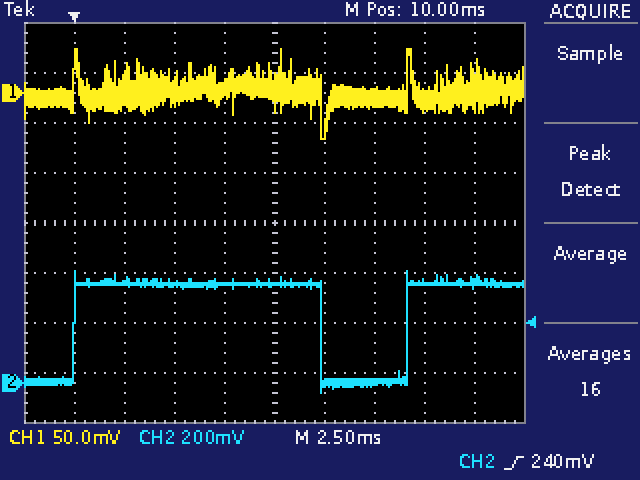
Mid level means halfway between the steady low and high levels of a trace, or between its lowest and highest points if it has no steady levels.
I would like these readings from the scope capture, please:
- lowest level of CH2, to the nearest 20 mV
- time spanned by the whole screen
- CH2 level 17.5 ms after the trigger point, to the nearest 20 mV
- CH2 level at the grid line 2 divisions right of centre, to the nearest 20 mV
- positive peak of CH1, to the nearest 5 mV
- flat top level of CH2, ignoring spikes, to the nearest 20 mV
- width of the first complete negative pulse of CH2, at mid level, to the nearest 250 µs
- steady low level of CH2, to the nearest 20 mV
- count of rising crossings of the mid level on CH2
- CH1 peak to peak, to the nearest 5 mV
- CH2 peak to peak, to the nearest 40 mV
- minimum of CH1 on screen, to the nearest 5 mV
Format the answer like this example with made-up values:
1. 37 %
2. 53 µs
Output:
1. -40 mV
2. 25 ms
3. 400 mV
4. 0 mV
5. 45 mV
6. 400 mV
7. 4.25 ms
8. 0 mV
9. 2
10. 90 mV
11. 480 mV
12. -45 mV
